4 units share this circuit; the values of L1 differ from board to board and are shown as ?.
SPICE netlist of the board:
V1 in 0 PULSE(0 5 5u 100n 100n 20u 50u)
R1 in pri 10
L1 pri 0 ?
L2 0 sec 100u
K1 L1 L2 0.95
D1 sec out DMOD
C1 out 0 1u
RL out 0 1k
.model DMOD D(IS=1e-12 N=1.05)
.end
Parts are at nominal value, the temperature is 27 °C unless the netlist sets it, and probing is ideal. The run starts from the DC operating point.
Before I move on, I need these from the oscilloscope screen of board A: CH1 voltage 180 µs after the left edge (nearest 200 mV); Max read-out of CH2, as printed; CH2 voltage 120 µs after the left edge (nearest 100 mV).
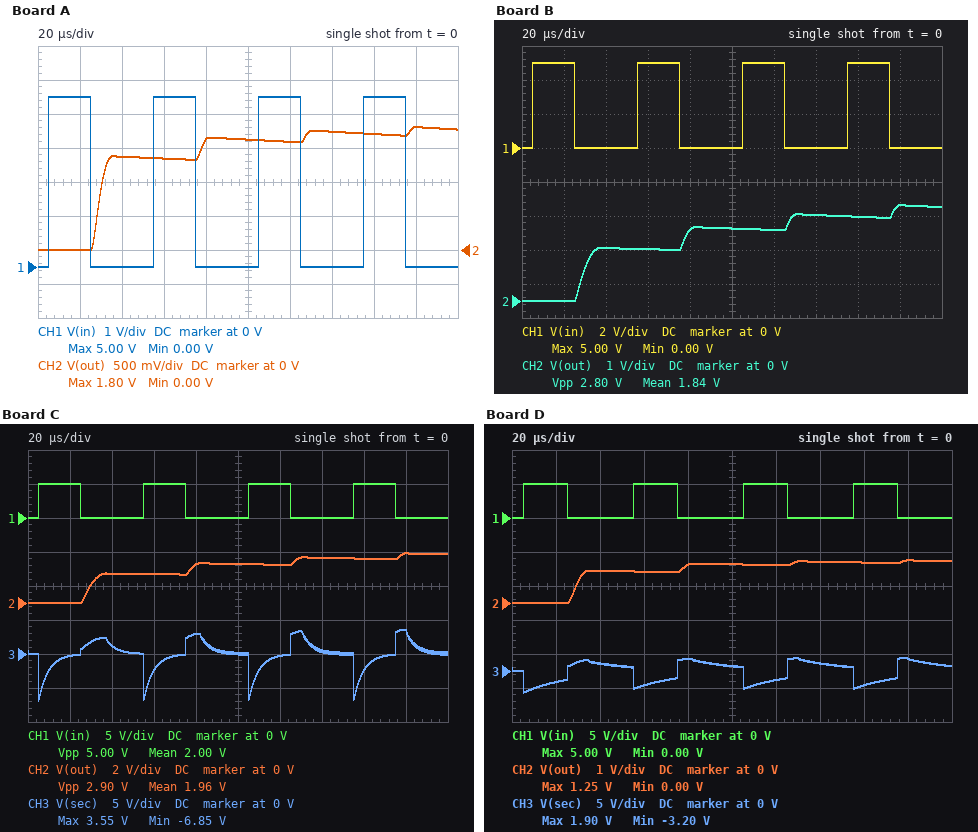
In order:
0 V
1.80 V
1.6 V
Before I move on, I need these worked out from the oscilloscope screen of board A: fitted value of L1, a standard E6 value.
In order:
150 µH
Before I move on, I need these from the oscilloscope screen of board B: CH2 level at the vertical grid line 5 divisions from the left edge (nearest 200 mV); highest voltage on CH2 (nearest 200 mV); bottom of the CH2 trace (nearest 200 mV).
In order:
2.2 V
2.8 V
0 V
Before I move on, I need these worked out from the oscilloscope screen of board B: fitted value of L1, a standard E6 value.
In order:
33 µH
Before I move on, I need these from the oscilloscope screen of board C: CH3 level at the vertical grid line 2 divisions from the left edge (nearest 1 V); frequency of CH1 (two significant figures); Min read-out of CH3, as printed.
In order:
1 V
20 kHz
-6.85 V
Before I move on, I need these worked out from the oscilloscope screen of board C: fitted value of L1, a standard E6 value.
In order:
47 µH
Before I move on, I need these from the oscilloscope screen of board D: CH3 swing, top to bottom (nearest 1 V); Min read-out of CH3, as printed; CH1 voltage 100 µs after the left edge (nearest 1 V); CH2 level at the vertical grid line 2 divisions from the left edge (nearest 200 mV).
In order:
5 V
-3.20 V
0 V
1.0 V
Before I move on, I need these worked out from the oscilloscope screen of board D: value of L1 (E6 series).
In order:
220 µH
